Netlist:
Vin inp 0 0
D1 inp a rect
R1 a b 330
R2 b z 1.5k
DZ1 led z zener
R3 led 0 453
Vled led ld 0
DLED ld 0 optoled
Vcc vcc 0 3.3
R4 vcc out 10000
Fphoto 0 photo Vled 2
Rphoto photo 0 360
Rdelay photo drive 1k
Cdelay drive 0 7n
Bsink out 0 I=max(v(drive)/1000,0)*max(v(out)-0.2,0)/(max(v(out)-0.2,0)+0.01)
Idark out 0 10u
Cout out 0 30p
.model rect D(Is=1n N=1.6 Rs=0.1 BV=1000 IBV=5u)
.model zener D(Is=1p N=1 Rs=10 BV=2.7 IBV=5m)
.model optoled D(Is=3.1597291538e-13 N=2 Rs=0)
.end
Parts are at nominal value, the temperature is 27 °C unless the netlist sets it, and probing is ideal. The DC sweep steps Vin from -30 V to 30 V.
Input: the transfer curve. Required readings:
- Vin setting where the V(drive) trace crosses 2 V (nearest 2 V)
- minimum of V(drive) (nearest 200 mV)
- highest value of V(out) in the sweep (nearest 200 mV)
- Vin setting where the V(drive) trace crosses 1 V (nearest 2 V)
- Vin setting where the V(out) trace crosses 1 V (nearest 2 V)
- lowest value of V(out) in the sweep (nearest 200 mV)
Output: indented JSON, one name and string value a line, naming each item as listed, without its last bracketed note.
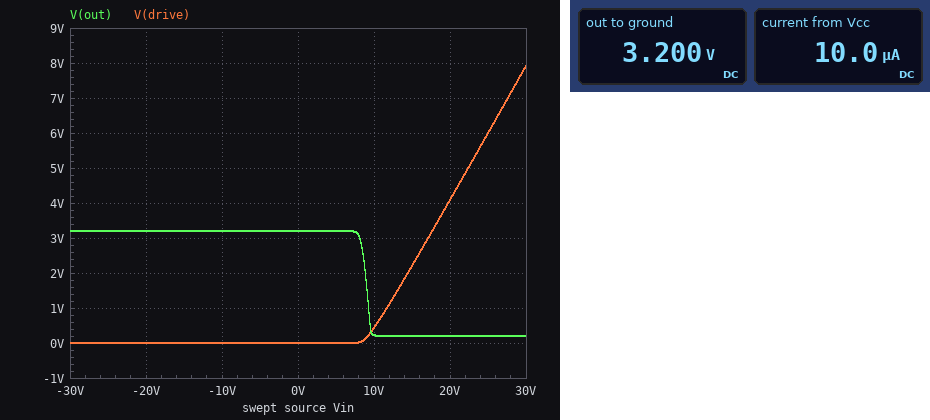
{
  "Vin setting where the V(drive) trace crosses 2 V": "14 V",
  "minimum of V(drive)": "0 V",
  "highest value of V(out) in the sweep": "3.2 V",
  "Vin setting where the V(drive) trace crosses 1 V": "12 V",
  "Vin setting where the V(out) trace crosses 1 V": "10 V",
  "lowest value of V(out) in the sweep": "200 mV"
}
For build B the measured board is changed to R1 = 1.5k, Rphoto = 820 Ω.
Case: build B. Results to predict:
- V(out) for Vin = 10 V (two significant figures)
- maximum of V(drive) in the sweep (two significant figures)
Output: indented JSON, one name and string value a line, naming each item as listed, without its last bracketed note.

{
  "V(out) for Vin = 10 V": "3.1 V",
  "maximum of V(drive) in the sweep": "9.4 V"
}
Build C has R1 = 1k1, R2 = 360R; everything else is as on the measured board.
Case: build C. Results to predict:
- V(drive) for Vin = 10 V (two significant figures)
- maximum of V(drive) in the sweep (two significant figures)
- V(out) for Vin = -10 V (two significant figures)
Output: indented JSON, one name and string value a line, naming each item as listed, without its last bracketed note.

{
  "V(drive) for Vin = 10 V": "900 mV",
  "maximum of V(drive) in the sweep": "10 V",
  "V(out) for Vin = -10 V": "3.2 V"
}
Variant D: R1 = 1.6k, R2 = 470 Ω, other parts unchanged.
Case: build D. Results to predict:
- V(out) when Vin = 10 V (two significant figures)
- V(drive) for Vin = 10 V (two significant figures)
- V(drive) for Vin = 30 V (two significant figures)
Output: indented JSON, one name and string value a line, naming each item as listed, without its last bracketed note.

{
  "V(out) when Vin = 10 V": "840 mV",
  "V(drive) for Vin = 10 V": "240 mV",
  "V(drive) for Vin = 30 V": "6.8 V"
}
